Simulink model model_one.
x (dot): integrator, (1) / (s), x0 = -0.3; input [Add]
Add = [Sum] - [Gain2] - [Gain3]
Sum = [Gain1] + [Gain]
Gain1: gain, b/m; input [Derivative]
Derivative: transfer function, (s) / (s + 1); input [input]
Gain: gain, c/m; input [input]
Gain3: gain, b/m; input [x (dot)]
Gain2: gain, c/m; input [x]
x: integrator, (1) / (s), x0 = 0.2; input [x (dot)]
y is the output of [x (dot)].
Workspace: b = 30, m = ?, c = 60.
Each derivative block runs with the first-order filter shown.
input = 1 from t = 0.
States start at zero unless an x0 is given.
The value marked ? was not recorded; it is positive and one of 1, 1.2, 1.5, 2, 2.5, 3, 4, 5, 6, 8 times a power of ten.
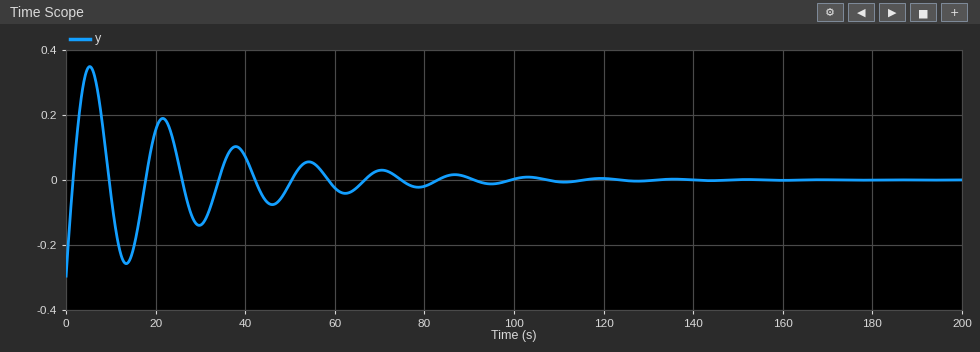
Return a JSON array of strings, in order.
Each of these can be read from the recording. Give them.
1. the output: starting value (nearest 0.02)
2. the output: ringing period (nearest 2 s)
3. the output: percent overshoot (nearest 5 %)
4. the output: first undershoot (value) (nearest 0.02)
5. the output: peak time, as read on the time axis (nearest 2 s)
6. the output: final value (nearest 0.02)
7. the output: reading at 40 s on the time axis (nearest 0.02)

["-0.30", "16 s", "115 %", "-0.26", "6 s", "0.00", "0.08"]
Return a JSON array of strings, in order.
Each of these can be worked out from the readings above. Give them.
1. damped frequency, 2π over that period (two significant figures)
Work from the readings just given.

["0.39 rad/s"]
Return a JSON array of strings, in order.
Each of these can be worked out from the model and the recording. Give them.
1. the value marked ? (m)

["400"]
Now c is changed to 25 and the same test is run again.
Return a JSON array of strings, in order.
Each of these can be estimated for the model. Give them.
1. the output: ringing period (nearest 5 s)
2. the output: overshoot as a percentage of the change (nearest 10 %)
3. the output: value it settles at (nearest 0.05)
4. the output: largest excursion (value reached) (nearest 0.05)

["25 s", "80 %", "0.00", "0.25"]
